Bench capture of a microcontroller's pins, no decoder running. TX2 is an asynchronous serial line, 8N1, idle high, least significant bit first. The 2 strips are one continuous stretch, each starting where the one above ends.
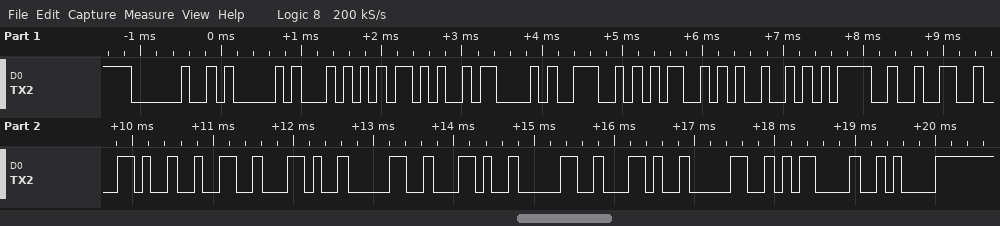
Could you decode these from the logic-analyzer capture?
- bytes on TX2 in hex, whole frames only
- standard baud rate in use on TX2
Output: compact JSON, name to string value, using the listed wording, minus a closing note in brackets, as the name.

{"bytes on TX2 in hex, whole frames only": "20 41 54 2B 43 4E 4D 49 3D 32 2C 32 2C 30 2C 30 2C 30 0D 0A", "standard baud rate in use on TX2": "9600 baud"}
